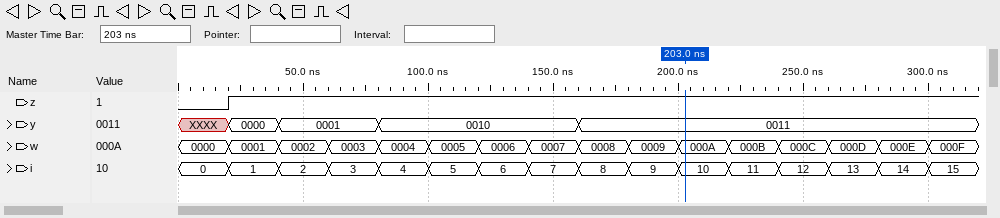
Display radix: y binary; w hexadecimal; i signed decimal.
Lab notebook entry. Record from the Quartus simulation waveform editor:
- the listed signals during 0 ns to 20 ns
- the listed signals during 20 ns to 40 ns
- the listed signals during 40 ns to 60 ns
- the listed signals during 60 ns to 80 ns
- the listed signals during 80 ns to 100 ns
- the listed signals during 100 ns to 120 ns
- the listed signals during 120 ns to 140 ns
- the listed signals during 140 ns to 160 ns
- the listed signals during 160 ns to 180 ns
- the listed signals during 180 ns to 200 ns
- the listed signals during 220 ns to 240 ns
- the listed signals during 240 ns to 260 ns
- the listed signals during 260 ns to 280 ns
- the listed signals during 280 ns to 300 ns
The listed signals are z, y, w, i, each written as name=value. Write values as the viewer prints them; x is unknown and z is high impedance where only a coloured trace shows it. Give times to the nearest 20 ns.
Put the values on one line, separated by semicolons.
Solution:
z=0, y=XXXX, w=0000, i=0; z=1, y=0000, w=0001, i=1; z=1, y=0001, w=0002, i=2; z=1, y=0001, w=0003, i=3; z=1, y=0010, w=0004, i=4; z=1, y=0010, w=0005, i=5; z=1, y=0010, w=0006, i=6; z=1, y=0010, w=0007, i=7; z=1, y=0011, w=0008, i=8; z=1, y=0011, w=0009, i=9; z=1, y=0011, w=000B, i=11; z=1, y=0011, w=000C, i=12; z=1, y=0011, w=000D, i=13; z=1, y=0011, w=000E, i=14
